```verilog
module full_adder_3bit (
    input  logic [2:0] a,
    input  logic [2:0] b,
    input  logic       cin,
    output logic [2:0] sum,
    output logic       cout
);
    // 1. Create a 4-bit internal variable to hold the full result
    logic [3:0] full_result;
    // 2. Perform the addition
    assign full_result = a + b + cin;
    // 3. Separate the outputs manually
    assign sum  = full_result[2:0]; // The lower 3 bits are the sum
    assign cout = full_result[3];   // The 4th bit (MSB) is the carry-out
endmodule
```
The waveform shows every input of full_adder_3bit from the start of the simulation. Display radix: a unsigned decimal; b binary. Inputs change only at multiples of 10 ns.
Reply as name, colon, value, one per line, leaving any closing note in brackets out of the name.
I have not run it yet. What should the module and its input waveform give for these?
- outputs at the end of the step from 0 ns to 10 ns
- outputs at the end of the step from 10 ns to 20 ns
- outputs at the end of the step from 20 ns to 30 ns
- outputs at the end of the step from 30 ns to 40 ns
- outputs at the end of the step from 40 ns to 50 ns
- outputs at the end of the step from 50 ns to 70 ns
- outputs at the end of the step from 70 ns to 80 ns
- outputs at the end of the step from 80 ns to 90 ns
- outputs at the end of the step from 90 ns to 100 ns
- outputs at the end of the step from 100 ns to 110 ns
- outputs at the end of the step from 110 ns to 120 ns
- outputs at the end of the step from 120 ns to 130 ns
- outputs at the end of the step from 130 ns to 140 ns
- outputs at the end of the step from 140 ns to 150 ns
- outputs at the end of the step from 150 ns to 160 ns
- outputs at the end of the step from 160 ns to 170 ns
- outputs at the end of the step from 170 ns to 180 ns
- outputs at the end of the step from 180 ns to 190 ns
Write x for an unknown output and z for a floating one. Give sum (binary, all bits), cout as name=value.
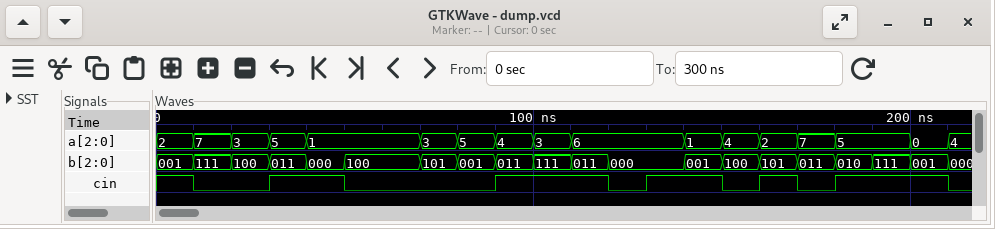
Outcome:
outputs at the end of the step from 0 ns to 10 ns: sum=100, cout=0
outputs at the end of the step from 10 ns to 20 ns: sum=110, cout=1
outputs at the end of the step from 20 ns to 30 ns: sum=111, cout=0
outputs at the end of the step from 30 ns to 40 ns: sum=001, cout=1
outputs at the end of the step from 40 ns to 50 ns: sum=010, cout=0
outputs at the end of the step from 50 ns to 70 ns: sum=101, cout=0
outputs at the end of the step from 70 ns to 80 ns: sum=000, cout=1
outputs at the end of the step from 80 ns to 90 ns: sum=110, cout=0
outputs at the end of the step from 90 ns to 100 ns: sum=000, cout=1
outputs at the end of the step from 100 ns to 110 ns: sum=011, cout=1
outputs at the end of the step from 110 ns to 120 ns: sum=010, cout=1
outputs at the end of the step from 120 ns to 130 ns: sum=110, cout=0
outputs at the end of the step from 130 ns to 140 ns: sum=111, cout=0
outputs at the end of the step from 140 ns to 150 ns: sum=011, cout=0
outputs at the end of the step from 150 ns to 160 ns: sum=000, cout=1
outputs at the end of the step from 160 ns to 170 ns: sum=000, cout=1
outputs at the end of the step from 170 ns to 180 ns: sum=010, cout=1
outputs at the end of the step from 180 ns to 190 ns: sum=000, cout=1
